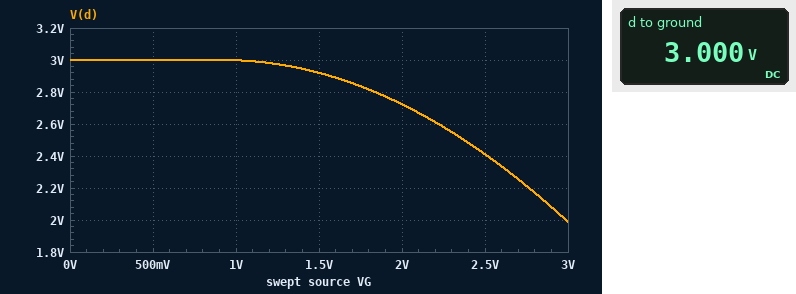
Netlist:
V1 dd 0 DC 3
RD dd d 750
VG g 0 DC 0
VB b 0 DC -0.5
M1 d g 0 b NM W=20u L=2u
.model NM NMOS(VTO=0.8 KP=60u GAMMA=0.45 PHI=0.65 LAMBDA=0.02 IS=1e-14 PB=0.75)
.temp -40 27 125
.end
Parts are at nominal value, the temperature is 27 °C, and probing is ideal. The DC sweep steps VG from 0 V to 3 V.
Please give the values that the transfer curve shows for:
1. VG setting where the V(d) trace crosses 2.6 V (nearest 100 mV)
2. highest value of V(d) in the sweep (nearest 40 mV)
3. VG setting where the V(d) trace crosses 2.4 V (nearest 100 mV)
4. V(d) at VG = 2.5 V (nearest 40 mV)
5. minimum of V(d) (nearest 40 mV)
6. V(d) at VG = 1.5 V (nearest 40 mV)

2.2 V
3.00 V
2.5 V
2.40 V
2.00 V
2.92 V
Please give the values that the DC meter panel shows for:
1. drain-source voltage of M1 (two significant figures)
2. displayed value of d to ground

3.0 V
3.000 V
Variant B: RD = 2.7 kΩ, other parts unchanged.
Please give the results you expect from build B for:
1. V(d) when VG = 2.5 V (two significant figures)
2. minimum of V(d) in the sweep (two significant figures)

1.1 V
800 mV
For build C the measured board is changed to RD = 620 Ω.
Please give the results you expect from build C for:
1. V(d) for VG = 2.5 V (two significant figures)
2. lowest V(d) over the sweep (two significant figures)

2.5 V
2.2 V
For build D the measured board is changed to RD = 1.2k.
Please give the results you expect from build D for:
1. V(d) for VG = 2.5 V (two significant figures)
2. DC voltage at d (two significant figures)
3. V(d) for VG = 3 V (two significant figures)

2.1 V
3.0 V
1.5 V
